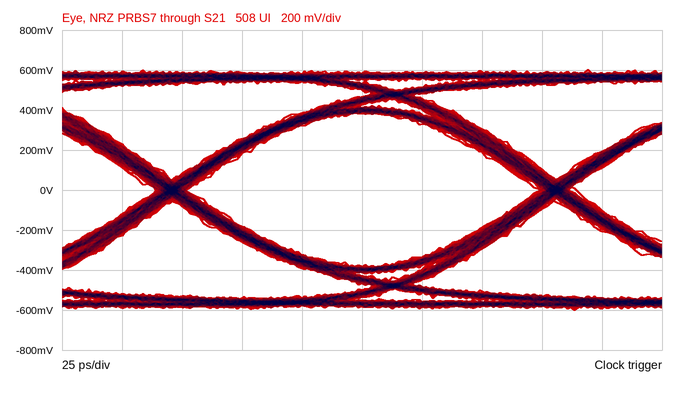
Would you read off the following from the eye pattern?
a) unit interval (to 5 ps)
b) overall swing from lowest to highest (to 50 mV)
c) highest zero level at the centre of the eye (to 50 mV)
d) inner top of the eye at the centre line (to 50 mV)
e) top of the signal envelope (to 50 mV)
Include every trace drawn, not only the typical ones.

160 ps
1.20 V
-400 mV
400 mV
600 mV
